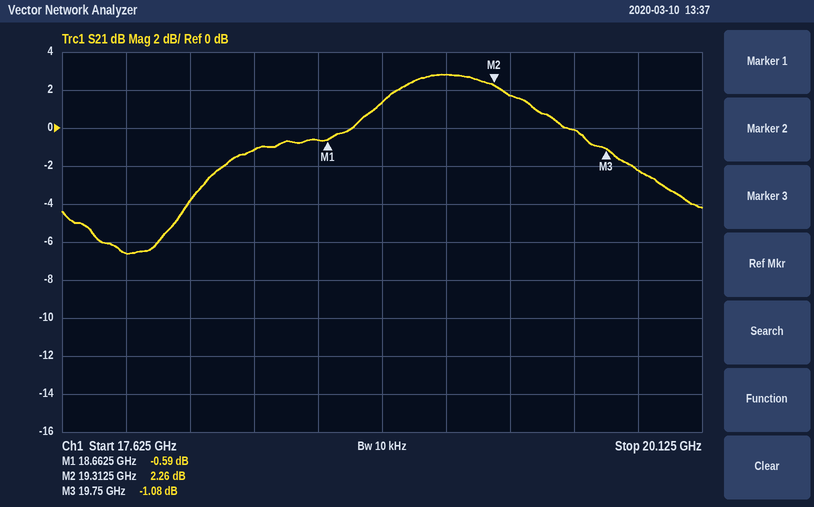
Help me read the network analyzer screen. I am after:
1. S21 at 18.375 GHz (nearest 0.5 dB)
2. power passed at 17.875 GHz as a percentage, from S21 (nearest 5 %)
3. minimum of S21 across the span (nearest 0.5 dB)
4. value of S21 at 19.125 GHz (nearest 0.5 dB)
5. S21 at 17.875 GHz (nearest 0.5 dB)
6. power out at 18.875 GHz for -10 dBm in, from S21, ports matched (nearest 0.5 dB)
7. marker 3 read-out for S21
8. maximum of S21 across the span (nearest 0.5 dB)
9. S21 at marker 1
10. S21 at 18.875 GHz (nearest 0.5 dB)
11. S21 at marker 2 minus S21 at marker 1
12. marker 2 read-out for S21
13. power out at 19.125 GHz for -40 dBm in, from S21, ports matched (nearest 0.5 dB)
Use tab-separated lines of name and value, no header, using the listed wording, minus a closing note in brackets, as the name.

S21 at 18.375 GHz	-1.0 dB
power passed at 17.875 GHz as a percentage, from S21	20 %
minimum of S21 across the span	-6.5 dB
value of S21 at 19.125 GHz	3.0 dB
S21 at 17.875 GHz	-6.5 dB
power out at 18.875 GHz for -10 dBm in, from S21, ports matched	-8.5 dBm
marker 3 read-out for S21	-1.08 dB
maximum of S21 across the span	3.0 dB
S21 at marker 1	-0.59 dB
S21 at 18.875 GHz	1.5 dB
S21 at marker 2 minus S21 at marker 1	2.85 dB
marker 2 read-out for S21	2.26 dB
power out at 19.125 GHz for -40 dBm in, from S21, ports matched	-37.0 dBm
